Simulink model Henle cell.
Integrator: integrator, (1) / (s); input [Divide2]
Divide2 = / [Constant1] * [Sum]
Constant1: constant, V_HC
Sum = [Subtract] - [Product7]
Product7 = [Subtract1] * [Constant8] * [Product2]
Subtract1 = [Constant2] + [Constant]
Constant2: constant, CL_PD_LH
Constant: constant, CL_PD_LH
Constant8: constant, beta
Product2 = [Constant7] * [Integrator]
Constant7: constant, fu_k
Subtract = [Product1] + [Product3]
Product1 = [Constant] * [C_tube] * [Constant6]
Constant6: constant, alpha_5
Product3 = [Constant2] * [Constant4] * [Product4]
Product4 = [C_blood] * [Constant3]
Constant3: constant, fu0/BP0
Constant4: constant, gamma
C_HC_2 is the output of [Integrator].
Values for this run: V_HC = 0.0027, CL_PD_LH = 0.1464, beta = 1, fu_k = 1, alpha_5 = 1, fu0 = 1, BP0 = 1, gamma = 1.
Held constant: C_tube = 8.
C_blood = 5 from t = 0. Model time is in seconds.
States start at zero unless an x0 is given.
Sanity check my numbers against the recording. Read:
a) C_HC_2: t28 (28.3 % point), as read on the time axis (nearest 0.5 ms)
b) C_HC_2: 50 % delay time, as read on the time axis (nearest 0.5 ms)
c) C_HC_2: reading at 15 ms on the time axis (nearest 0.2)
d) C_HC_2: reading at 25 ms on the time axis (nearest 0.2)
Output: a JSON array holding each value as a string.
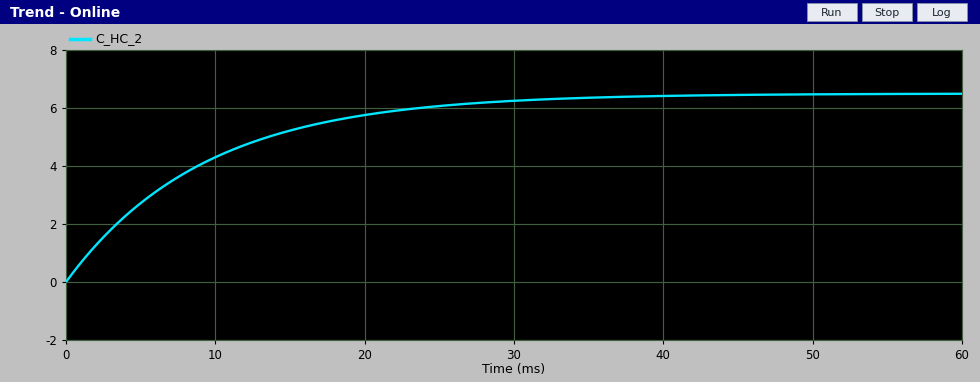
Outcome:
["3.0 ms", "6.5 ms", "5.2", "6.0"]
